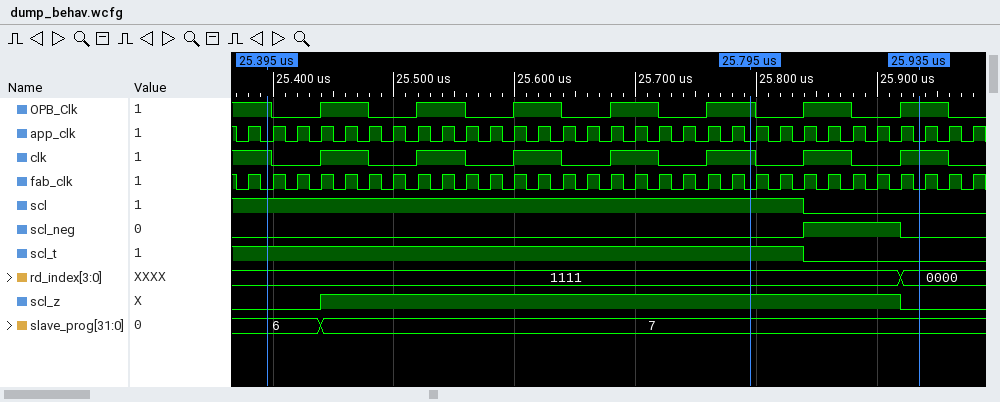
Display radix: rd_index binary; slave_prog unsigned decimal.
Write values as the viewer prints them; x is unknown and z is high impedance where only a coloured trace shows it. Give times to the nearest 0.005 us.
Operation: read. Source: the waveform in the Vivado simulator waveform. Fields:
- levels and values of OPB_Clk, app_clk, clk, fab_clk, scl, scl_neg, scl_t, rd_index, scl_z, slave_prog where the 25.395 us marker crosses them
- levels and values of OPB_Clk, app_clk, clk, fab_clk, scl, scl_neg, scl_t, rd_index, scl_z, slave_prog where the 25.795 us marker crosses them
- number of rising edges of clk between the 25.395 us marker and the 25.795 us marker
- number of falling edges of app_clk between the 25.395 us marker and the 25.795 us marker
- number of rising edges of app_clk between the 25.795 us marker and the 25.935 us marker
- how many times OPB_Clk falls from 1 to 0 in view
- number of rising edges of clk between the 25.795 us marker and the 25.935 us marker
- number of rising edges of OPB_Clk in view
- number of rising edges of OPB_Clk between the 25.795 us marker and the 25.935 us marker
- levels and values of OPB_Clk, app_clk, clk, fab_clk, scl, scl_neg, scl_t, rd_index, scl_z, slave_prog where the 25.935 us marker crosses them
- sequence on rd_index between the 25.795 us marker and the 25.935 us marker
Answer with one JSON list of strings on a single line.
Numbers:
["OPB_Clk=1, app_clk=0, clk=1, fab_clk=0, scl=1, scl_neg=0, scl_t=1, rd_index=1111, scl_z=0, slave_prog=6", "OPB_Clk=1, app_clk=0, clk=1, fab_clk=0, scl=1, scl_neg=0, scl_t=1, rd_index=1111, scl_z=1, slave_prog=7", "5", "20", "7", "8", "2", "7", "2", "OPB_Clk=1, app_clk=0, clk=1, fab_clk=0, scl=0, scl_neg=0, scl_t=0, rd_index=0000, scl_z=0, slave_prog=7", "1111, 0000"]
